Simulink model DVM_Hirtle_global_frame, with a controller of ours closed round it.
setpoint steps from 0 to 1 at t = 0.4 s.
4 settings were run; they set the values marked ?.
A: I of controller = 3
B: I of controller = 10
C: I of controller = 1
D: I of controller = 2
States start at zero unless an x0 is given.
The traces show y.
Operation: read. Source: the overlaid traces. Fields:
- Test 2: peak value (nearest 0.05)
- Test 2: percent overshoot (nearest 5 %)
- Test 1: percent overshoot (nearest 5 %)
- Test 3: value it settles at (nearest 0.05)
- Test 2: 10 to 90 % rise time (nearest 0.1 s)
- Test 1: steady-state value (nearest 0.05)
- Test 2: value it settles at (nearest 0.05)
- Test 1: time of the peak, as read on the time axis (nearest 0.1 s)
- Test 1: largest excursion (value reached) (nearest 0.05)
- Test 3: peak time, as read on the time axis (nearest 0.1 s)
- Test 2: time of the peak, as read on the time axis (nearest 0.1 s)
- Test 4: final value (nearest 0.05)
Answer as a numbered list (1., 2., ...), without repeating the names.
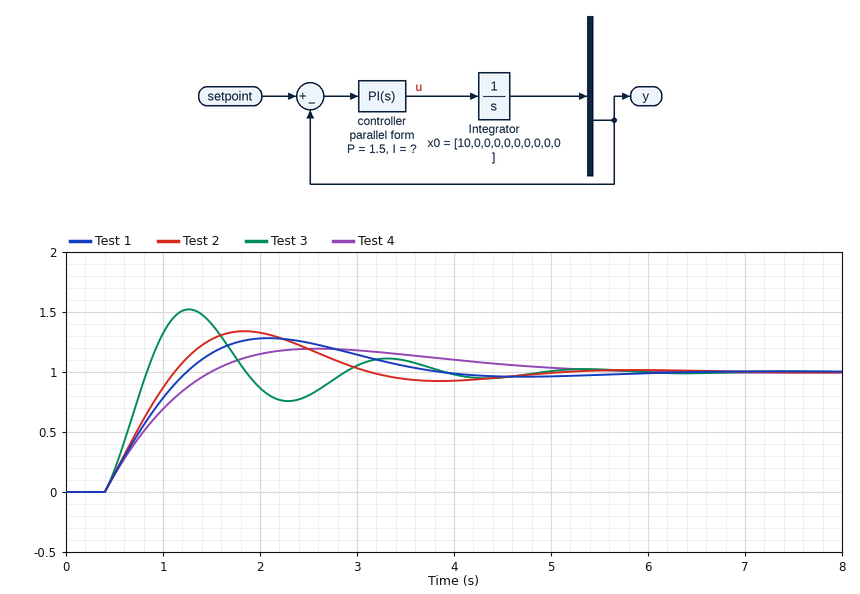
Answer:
1. 1.35
2. 35 %
3. 30 %
4. 1.00
5. 0.6 s
6. 1.00
7. 1.00
8. 2.1 s
9. 1.30
10. 1.3 s
11. 1.8 s
12. 1.00
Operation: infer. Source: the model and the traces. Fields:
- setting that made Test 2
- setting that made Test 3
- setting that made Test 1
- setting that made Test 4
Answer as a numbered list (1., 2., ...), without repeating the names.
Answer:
1. A
2. B
3. D
4. C
